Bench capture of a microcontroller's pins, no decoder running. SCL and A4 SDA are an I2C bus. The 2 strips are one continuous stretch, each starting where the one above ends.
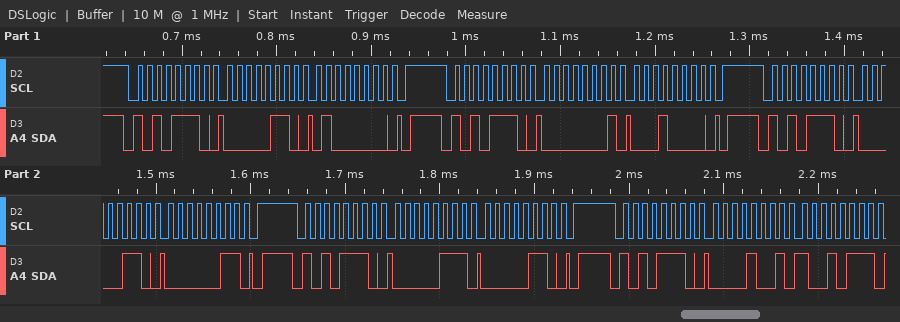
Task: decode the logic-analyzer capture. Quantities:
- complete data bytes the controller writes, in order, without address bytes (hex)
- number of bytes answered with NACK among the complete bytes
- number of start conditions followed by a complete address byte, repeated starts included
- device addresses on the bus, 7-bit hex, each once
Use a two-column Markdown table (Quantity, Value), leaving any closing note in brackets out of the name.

| Quantity | Value |
|---|---|
| complete data bytes the controller writes, in order, without address bytes | 06 40 01 10 06 03 07 06 09 97 |
| number of bytes answered with NACK among the complete bytes | 0 |
| number of start conditions followed by a complete address byte, repeated starts included | 5 |
| device addresses on the bus, 7-bit hex, each once | 0x57 |
